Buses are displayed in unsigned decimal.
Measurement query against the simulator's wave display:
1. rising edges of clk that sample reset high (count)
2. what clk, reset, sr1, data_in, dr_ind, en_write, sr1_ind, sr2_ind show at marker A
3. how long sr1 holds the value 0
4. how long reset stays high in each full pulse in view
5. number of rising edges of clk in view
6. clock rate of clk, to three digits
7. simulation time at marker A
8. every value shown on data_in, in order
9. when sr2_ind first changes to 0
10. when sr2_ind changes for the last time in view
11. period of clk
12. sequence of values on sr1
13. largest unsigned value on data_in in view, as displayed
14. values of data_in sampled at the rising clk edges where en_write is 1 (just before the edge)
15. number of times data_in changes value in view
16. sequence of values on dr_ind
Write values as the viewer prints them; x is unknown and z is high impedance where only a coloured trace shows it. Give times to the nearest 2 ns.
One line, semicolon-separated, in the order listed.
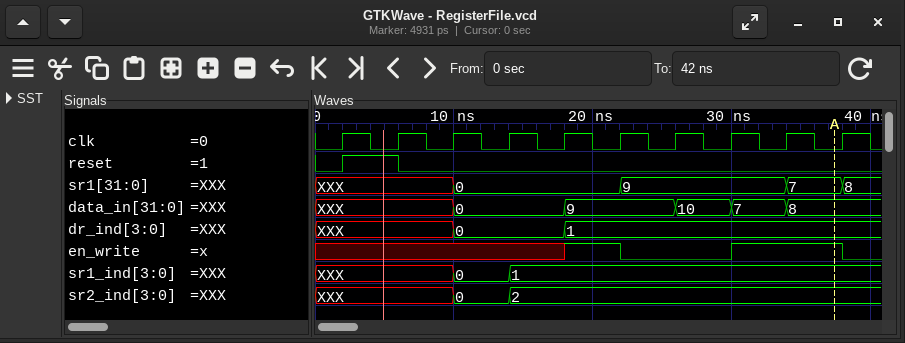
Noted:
1; clk=0, reset=0, sr1=7, data_in=8, dr_ind=1, en_write=1, sr1_ind=1, sr2_ind=2; 12 ns; 4 ns; 10; 250 MHz; 38 ns; XXX, 0, 9, 10, 7, 8; 10 ns; 14 ns; 4 ns; XXX, 0, 9, 7, 8; 10; 9, 7, 8; 5; XXX, 0, 1
